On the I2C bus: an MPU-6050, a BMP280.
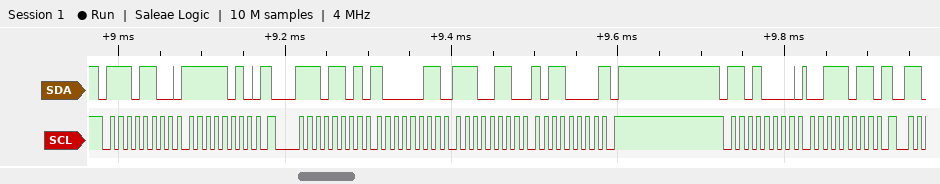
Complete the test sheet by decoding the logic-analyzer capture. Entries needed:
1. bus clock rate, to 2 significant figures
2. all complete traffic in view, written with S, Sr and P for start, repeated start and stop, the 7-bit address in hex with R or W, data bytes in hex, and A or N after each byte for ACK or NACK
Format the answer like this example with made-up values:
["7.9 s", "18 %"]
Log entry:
["100 kHz", "S 76W A FA A Sr 76R A 83 A E6 A B0 N P S 68W A 3B A"]
